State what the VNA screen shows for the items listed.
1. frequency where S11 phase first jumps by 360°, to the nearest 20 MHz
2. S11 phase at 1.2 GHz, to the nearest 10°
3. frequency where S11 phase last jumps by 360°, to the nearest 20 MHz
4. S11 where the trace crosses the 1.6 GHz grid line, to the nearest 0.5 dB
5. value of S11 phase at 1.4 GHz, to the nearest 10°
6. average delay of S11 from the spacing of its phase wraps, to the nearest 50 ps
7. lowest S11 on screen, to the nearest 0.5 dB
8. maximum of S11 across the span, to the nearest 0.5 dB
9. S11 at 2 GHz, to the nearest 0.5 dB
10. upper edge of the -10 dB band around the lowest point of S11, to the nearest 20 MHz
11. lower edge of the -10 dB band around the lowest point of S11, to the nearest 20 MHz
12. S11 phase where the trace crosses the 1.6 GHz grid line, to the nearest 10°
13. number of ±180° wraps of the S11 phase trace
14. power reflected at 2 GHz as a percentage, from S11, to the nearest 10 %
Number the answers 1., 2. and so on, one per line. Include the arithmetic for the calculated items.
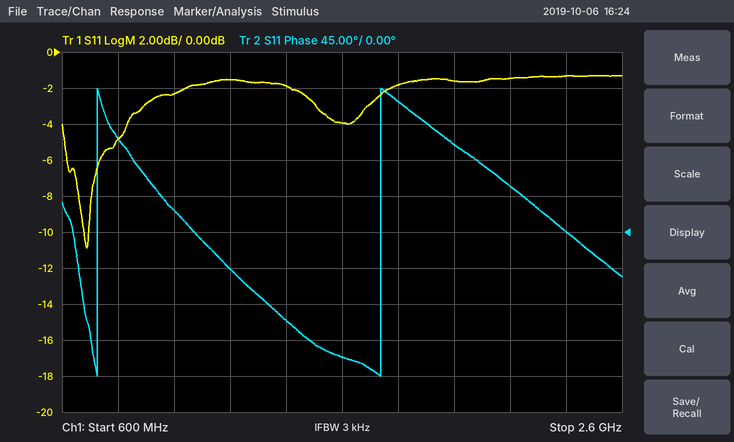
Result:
1. 720 MHz
2. -50°
3. 1.74 GHz
4. -4.0 dB
5. -110°
6. 1 cycle / (1.74 GHz − 720 MHz) ≈ 0.980 ns, so 1.00 ns to the nearest 50 ps
7. -11.0 dB
8. -1.5 dB
9. -1.5 dB
10. 700 MHz
11. 680 MHz
12. -160°
13. 2
14. 10^(-1.5/10) ≈ 70.8 %, so 70 % to the nearest 10 %
